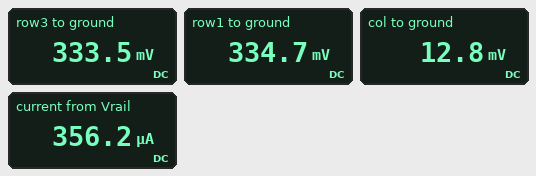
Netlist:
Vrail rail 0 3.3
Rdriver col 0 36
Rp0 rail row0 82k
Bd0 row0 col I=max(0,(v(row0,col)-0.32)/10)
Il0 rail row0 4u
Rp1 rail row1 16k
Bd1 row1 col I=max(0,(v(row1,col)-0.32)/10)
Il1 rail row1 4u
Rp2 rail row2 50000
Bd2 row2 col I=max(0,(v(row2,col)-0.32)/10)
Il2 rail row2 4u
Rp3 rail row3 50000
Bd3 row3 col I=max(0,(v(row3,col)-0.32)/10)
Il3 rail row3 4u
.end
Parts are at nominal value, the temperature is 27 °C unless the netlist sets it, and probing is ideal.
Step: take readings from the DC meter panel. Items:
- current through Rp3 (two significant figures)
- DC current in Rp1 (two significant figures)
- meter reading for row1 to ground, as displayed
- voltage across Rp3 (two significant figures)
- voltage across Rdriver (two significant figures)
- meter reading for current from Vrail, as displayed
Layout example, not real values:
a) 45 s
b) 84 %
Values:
a) 59 µA
b) 190 µA
c) 334.7 mV
d) 3.0 V
e) 13 mV
f) 356.2 µA
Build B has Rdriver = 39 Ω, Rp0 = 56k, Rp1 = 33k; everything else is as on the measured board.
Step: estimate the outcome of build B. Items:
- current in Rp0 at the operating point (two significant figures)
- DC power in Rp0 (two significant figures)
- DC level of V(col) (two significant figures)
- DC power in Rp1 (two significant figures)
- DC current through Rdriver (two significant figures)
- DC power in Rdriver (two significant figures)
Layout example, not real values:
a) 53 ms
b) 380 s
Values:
a) 53 µA
b) 160 µW
c) 11 mV
d) 270 µW
e) 280 µA
f) 3.0 µW
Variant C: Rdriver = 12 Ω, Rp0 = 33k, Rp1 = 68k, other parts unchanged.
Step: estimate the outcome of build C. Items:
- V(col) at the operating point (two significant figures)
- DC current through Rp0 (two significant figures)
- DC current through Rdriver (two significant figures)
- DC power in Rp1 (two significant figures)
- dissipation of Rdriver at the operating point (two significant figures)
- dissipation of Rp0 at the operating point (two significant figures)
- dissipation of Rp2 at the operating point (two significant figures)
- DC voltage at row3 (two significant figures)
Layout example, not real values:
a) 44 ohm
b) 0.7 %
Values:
a) 3.2 mV
b) 90 µA
c) 270 µA
d) 130 µW
e) 870 nW
f) 270 µW
g) 180 µW
h) 320 mV
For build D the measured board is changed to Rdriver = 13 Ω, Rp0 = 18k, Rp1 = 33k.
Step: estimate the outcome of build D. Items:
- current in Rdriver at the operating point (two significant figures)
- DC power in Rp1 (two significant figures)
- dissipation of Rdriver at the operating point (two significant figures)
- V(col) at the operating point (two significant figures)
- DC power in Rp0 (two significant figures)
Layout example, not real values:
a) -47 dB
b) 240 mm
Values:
a) 390 µA
b) 270 µW
c) 2.0 µW
d) 5.1 mV
e) 490 µW
